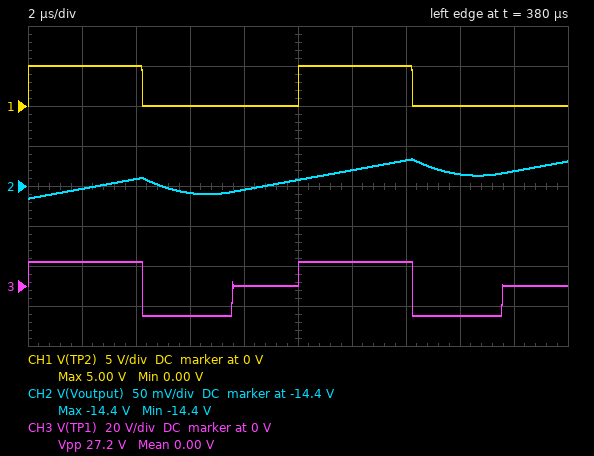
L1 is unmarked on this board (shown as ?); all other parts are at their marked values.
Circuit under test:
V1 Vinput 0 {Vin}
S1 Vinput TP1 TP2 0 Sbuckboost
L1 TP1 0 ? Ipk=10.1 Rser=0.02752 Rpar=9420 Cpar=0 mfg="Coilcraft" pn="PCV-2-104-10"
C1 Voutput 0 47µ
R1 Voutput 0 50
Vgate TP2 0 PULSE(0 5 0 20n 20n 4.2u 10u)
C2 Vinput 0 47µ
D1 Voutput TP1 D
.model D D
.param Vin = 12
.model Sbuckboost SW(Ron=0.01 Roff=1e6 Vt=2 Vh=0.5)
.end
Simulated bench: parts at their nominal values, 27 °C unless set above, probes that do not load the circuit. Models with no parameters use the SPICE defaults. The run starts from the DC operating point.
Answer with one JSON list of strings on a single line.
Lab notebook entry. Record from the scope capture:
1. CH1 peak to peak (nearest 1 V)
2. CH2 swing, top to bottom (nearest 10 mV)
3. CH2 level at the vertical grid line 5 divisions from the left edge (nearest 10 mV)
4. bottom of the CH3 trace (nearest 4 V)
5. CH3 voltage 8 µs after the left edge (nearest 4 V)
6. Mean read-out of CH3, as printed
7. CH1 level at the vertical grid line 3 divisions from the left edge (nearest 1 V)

["5 V", "50 mV", "-14.39 V", "-16 V", "0 V", "0.00 V", "0 V"]
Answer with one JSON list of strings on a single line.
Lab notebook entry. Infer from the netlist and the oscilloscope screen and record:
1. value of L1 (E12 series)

["47 µH"]
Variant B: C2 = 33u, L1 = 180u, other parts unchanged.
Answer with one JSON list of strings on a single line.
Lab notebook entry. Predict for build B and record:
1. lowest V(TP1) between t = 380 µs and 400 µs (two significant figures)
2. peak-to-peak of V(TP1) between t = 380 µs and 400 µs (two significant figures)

["-14 V", "26 V"]
